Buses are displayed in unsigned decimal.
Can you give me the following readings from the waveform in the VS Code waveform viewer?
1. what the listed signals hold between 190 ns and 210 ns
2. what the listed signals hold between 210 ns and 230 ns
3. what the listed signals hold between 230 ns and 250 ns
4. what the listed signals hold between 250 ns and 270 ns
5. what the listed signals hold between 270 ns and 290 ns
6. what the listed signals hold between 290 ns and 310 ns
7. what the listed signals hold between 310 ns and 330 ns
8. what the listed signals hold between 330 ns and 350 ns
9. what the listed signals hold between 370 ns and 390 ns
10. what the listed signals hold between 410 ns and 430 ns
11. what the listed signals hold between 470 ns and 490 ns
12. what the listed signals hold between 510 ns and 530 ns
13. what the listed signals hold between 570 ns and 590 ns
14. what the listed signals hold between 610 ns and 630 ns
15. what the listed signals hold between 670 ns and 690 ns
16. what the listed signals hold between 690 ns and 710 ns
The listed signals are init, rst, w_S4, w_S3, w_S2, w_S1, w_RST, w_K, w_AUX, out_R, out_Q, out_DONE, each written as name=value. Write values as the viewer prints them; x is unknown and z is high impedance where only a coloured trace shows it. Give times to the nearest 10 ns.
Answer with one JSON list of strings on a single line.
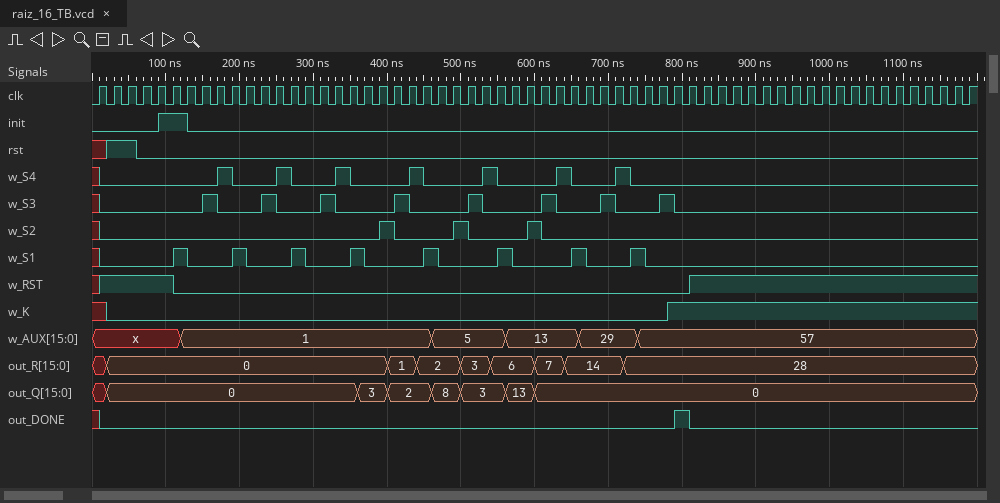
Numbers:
["init=0, rst=0, w_S4=0, w_S3=0, w_S2=0, w_S1=1, w_RST=0, w_K=0, w_AUX=1, out_R=0, out_Q=0, out_DONE=0", "init=0, rst=0, w_S4=0, w_S3=0, w_S2=0, w_S1=0, w_RST=0, w_K=0, w_AUX=1, out_R=0, out_Q=0, out_DONE=0", "init=0, rst=0, w_S4=0, w_S3=1, w_S2=0, w_S1=0, w_RST=0, w_K=0, w_AUX=1, out_R=0, out_Q=0, out_DONE=0", "init=0, rst=0, w_S4=1, w_S3=0, w_S2=0, w_S1=0, w_RST=0, w_K=0, w_AUX=1, out_R=0, out_Q=0, out_DONE=0", "init=0, rst=0, w_S4=0, w_S3=0, w_S2=0, w_S1=1, w_RST=0, w_K=0, w_AUX=1, out_R=0, out_Q=0, out_DONE=0", "init=0, rst=0, w_S4=0, w_S3=0, w_S2=0, w_S1=0, w_RST=0, w_K=0, w_AUX=1, out_R=0, out_Q=0, out_DONE=0", "init=0, rst=0, w_S4=0, w_S3=1, w_S2=0, w_S1=0, w_RST=0, w_K=0, w_AUX=1, out_R=0, out_Q=0, out_DONE=0", "init=0, rst=0, w_S4=1, w_S3=0, w_S2=0, w_S1=0, w_RST=0, w_K=0, w_AUX=1, out_R=0, out_Q=0, out_DONE=0", "init=0, rst=0, w_S4=0, w_S3=0, w_S2=0, w_S1=0, w_RST=0, w_K=0, w_AUX=1, out_R=0, out_Q=3, out_DONE=0", "init=0, rst=0, w_S4=0, w_S3=1, w_S2=0, w_S1=0, w_RST=0, w_K=0, w_AUX=1, out_R=1, out_Q=2, out_DONE=0", "init=0, rst=0, w_S4=0, w_S3=0, w_S2=0, w_S1=0, w_RST=0, w_K=0, w_AUX=5, out_R=2, out_Q=8, out_DONE=0", "init=0, rst=0, w_S4=0, w_S3=1, w_S2=0, w_S1=0, w_RST=0, w_K=0, w_AUX=5, out_R=3, out_Q=3, out_DONE=0", "init=0, rst=0, w_S4=0, w_S3=0, w_S2=0, w_S1=0, w_RST=0, w_K=0, w_AUX=13, out_R=6, out_Q=13, out_DONE=0", "init=0, rst=0, w_S4=0, w_S3=1, w_S2=0, w_S1=0, w_RST=0, w_K=0, w_AUX=13, out_R=7, out_Q=0, out_DONE=0", "init=0, rst=0, w_S4=0, w_S3=0, w_S2=0, w_S1=0, w_RST=0, w_K=0, w_AUX=29, out_R=14, out_Q=0, out_DONE=0", "init=0, rst=0, w_S4=0, w_S3=1, w_S2=0, w_S1=0, w_RST=0, w_K=0, w_AUX=29, out_R=14, out_Q=0, out_DONE=0"]
